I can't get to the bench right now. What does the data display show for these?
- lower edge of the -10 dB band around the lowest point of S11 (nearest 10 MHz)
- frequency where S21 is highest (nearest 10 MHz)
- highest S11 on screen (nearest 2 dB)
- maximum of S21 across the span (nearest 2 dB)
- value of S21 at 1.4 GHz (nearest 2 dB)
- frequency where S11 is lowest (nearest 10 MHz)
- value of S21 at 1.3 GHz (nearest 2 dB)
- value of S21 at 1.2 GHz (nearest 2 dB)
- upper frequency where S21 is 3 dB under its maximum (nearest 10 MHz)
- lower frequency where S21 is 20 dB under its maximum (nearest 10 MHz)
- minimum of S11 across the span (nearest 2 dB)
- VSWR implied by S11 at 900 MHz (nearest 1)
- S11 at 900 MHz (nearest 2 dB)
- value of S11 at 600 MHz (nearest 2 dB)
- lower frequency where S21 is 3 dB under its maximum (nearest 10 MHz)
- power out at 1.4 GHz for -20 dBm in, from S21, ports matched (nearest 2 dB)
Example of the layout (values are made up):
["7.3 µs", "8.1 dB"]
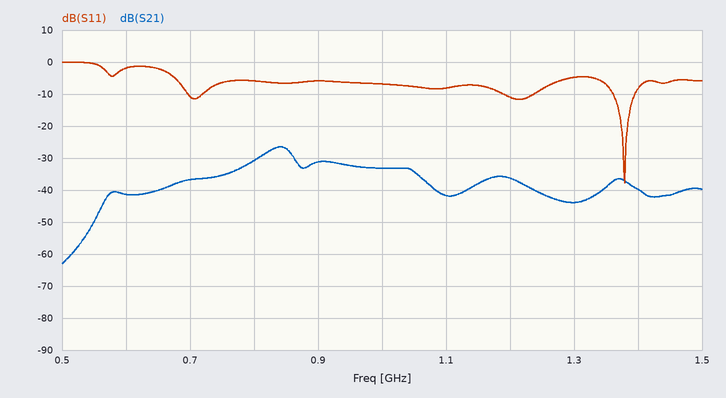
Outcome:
["1.36 GHz", "840 MHz", "0 dB", "-26 dB", "-40 dB", "1.38 GHz", "-44 dB", "-36 dB", "860 MHz", "560 MHz", "-38 dB", "3", "-6 dB", "-2 dB", "810 MHz", "-60 dBm"]
